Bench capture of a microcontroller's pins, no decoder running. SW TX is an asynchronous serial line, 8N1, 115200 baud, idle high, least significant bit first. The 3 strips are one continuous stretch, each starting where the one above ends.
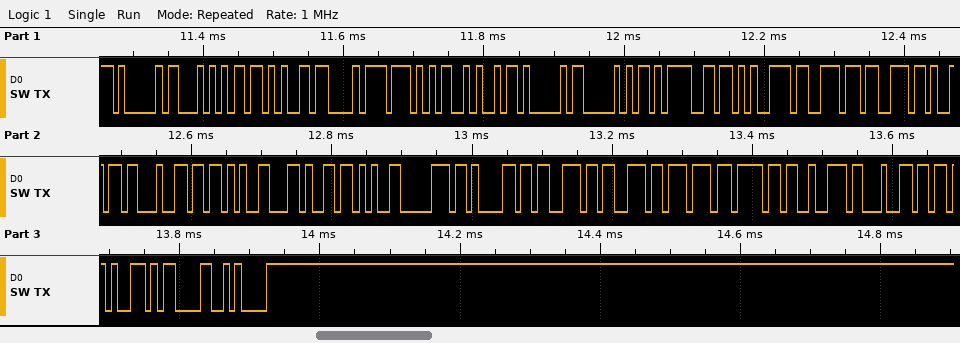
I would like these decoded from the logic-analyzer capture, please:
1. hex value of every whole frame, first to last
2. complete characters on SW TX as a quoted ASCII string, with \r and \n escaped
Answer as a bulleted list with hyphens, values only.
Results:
- 41 54 2B 43 57 4A 41 50 3D 2B 73 73 69 64 2B 2C 2B 70 61 73 73 77 6F 72 64 2B 0D 0A
- "AT+CWJAP=+ssid+,+password+\r\n"
